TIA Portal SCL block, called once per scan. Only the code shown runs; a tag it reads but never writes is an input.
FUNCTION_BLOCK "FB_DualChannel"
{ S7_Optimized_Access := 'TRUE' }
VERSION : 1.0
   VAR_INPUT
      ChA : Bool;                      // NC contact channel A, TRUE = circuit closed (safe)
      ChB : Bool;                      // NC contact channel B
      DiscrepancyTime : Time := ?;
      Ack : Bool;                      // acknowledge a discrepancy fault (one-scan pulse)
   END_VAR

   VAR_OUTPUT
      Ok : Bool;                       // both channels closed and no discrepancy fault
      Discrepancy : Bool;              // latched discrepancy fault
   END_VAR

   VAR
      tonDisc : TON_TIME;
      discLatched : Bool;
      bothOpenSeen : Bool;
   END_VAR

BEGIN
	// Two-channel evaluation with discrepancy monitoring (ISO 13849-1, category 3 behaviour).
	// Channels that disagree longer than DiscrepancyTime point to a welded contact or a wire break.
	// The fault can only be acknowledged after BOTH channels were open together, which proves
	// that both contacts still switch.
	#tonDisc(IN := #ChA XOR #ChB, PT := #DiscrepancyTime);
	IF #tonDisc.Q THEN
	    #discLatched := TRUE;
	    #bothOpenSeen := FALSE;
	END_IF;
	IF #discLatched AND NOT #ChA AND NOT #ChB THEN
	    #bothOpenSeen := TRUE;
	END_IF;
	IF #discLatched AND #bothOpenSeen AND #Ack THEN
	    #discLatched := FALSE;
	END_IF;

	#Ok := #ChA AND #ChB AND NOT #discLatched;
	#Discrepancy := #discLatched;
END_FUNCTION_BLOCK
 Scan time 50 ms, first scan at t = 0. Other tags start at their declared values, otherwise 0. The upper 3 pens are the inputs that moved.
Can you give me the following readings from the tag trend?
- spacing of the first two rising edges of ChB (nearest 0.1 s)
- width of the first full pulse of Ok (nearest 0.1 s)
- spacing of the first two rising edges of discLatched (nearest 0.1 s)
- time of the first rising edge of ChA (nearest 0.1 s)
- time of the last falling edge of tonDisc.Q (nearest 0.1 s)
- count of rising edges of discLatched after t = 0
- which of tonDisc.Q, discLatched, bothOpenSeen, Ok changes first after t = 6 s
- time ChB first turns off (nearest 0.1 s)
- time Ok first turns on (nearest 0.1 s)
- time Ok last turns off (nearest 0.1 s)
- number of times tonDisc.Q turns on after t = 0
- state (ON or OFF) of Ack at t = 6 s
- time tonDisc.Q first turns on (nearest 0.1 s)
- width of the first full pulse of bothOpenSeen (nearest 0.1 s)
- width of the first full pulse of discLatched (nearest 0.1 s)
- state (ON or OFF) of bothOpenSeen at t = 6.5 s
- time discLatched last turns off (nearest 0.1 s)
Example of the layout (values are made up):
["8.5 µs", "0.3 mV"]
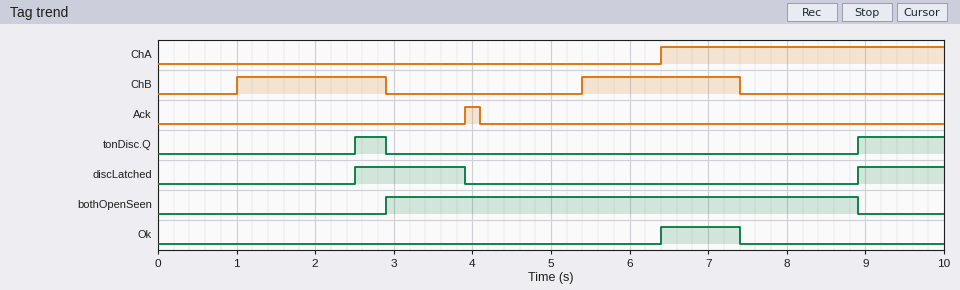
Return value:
["4.4 s", "1.0 s", "6.4 s", "6.4 s", "2.9 s", "2", "Ok", "2.9 s", "6.4 s", "7.4 s", "2", "OFF", "2.5 s", "6.0 s", "1.4 s", "ON", "3.9 s"]
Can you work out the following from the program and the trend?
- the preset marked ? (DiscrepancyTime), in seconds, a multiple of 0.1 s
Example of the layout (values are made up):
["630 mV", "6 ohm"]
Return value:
["1.5 s"]
